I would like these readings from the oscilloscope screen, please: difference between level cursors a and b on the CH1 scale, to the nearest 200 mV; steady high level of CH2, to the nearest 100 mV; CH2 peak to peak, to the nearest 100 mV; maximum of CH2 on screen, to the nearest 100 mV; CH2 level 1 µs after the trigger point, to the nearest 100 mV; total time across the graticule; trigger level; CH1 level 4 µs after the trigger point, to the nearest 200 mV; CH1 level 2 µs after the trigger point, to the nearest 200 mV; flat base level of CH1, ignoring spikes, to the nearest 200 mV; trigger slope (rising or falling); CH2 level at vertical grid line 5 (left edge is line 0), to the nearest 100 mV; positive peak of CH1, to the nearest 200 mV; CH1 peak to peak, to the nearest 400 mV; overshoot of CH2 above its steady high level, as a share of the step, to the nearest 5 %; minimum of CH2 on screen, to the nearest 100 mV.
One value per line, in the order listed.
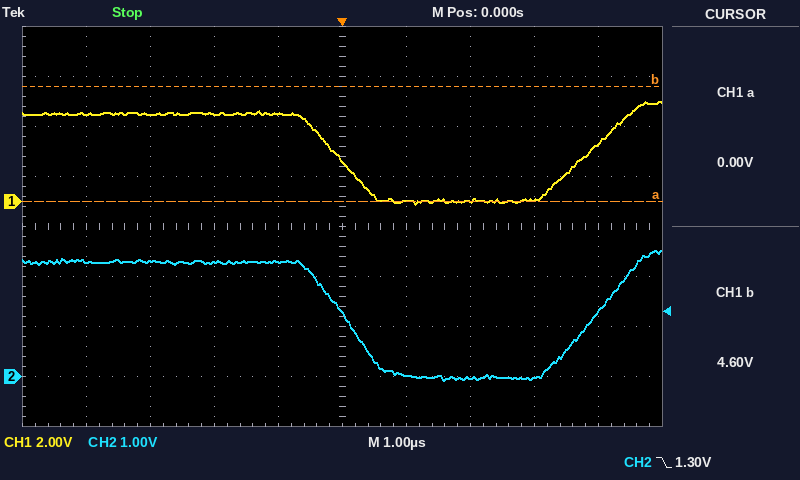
4.6 V
2.3 V
2.6 V
2.5 V
0.0 V
10 µs
1.30 V
2.4 V
0.0 V
0.0 V
falling
1.3 V
4.0 V
4.0 V
10 %
-100 mV
